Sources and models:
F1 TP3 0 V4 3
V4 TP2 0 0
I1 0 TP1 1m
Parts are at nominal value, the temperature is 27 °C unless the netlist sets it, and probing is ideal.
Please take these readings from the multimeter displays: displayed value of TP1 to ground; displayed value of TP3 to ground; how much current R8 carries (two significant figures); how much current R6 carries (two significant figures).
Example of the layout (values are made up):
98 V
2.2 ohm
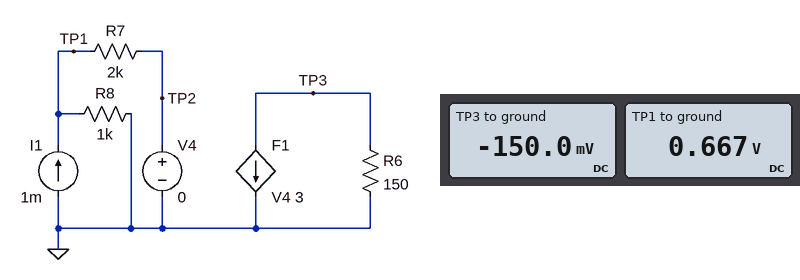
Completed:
0.667 V
-150.0 mV
670 µA
1.0 mA
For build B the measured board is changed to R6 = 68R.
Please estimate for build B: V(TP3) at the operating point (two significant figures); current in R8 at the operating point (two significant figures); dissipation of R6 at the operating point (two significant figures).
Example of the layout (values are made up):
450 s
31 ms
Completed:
-68 mV
670 µA
68 µW
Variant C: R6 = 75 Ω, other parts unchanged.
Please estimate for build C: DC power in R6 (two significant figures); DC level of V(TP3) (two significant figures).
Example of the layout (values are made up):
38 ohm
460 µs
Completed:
75 µW
-75 mV
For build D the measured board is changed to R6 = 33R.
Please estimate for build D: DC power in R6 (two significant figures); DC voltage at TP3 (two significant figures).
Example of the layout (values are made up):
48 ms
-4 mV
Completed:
33 µW
-33 mV
